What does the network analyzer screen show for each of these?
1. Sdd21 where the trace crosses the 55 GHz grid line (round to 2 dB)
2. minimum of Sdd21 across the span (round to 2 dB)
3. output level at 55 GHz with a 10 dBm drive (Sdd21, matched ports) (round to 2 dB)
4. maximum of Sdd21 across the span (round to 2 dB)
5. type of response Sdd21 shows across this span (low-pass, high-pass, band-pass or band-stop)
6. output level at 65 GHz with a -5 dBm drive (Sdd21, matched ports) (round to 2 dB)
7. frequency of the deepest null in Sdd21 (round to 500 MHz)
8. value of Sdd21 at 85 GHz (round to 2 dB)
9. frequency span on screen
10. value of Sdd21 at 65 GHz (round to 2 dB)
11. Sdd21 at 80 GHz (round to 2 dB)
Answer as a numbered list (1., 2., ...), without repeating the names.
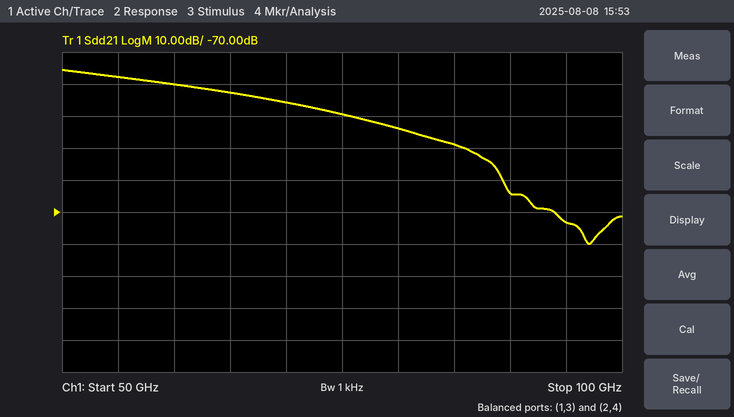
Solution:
1. -28 dB
2. -80 dB
3. -18 dBm
4. -26 dB
5. low-pass
6. -38 dBm
7. 97.0 GHz
8. -48 dB
9. 50 GHz
10. -32 dB
11. -44 dB
